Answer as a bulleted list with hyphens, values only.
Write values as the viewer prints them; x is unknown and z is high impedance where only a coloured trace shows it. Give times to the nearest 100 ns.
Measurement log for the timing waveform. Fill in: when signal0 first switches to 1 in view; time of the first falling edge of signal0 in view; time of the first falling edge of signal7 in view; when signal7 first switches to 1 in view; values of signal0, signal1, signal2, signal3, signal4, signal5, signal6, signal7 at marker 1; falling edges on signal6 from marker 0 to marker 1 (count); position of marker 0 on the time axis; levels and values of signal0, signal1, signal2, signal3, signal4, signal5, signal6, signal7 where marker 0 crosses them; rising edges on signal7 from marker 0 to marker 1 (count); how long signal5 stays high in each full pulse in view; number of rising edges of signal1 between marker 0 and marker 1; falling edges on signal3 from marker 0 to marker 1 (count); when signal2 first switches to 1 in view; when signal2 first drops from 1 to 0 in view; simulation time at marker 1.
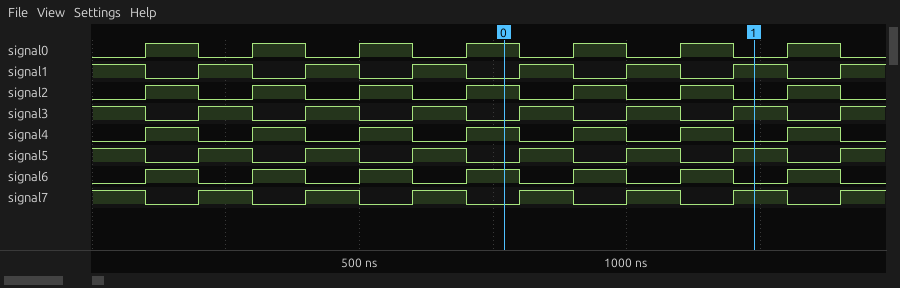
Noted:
- 100 ns
- 200 ns
- 100 ns
- 200 ns
- signal0=0, signal1=1, signal2=0, signal3=1, signal4=0, signal5=1, signal6=0, signal7=1
- 3
- 800 ns
- signal0=1, signal1=0, signal2=1, signal3=0, signal4=1, signal5=0, signal6=1, signal7=0
- 3
- 100 ns, 100 ns, 100 ns, 100 ns, 100 ns, 100 ns
- 3
- 2
- 100 ns
- 200 ns
- 1200 ns
